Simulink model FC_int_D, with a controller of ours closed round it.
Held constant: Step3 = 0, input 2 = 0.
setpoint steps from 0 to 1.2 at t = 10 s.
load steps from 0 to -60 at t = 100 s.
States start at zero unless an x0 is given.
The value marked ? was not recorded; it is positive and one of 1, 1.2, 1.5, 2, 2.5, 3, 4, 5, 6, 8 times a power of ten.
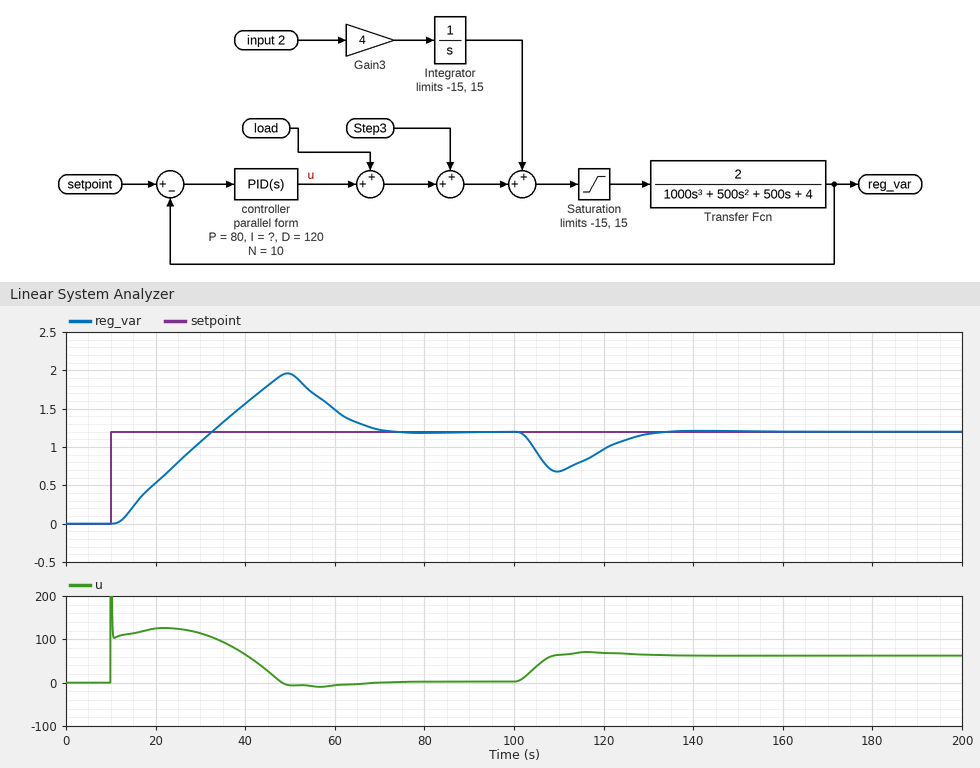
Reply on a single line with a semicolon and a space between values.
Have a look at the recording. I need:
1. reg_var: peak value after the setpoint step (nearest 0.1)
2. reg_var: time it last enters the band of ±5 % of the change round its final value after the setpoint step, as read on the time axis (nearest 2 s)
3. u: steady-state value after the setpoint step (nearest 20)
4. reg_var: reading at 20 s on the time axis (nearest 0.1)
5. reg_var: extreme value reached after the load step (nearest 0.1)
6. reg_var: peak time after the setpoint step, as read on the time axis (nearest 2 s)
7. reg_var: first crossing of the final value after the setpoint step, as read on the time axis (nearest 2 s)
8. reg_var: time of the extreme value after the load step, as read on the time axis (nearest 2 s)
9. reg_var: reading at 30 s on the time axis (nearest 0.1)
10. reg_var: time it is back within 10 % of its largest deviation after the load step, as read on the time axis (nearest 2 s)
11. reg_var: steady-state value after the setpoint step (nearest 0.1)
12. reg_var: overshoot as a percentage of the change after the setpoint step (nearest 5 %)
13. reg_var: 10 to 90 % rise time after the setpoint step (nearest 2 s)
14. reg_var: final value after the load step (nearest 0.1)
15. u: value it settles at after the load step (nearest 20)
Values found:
2.0; 68 s; 0; 0.5; 0.7; 50 s; 32 s; 110 s; 1.1; 128 s; 1.2; 65 %; 16 s; 1.2; 60
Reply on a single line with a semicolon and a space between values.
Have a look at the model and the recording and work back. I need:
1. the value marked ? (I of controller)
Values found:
8
